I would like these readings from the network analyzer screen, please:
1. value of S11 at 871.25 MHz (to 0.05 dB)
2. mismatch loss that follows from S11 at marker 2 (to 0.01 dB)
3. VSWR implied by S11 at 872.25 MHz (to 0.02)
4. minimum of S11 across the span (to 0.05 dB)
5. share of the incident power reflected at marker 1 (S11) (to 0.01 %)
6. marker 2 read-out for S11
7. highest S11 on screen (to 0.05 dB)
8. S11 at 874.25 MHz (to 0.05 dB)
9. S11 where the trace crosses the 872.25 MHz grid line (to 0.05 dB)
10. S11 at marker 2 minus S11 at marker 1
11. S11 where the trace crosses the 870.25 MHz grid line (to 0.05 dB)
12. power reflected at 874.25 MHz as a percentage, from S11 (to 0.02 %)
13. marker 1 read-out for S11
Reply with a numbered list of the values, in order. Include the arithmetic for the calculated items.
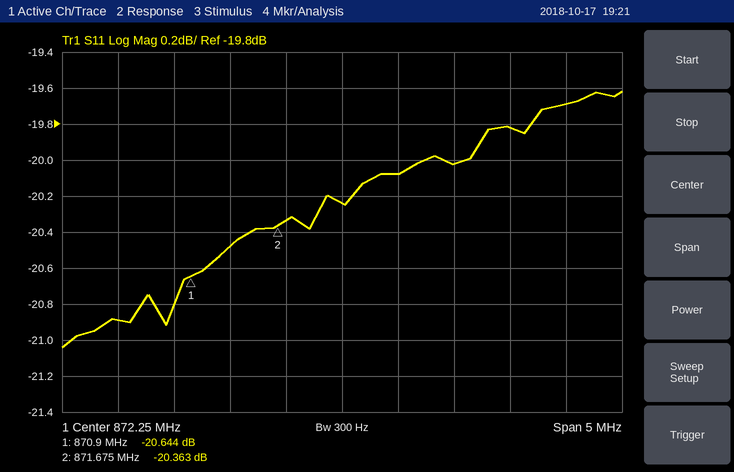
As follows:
1. -20.50 dB
2. −10 log10(1 − 10^(-20.363/10)) ≈ 0.04 dB
3. |Γ| = 10^(-20.25/20) = 0.0972; VSWR = (1 + 0.0972)/(1 − 0.0972) ≈ 1.22
4. -21.05 dB
5. 10^(-20.644/10) ≈ 0.86 %
6. -20.363 dB
7. -19.60 dB
8. -19.70 dB
9. -20.25 dB
10. -20.363 − (-20.644) = 0.281 dB
11. -20.90 dB
12. 10^(-19.7/10) ≈ 1.07 %, so 1.08 % to the nearest 0.02 %
13. -20.644 dB
